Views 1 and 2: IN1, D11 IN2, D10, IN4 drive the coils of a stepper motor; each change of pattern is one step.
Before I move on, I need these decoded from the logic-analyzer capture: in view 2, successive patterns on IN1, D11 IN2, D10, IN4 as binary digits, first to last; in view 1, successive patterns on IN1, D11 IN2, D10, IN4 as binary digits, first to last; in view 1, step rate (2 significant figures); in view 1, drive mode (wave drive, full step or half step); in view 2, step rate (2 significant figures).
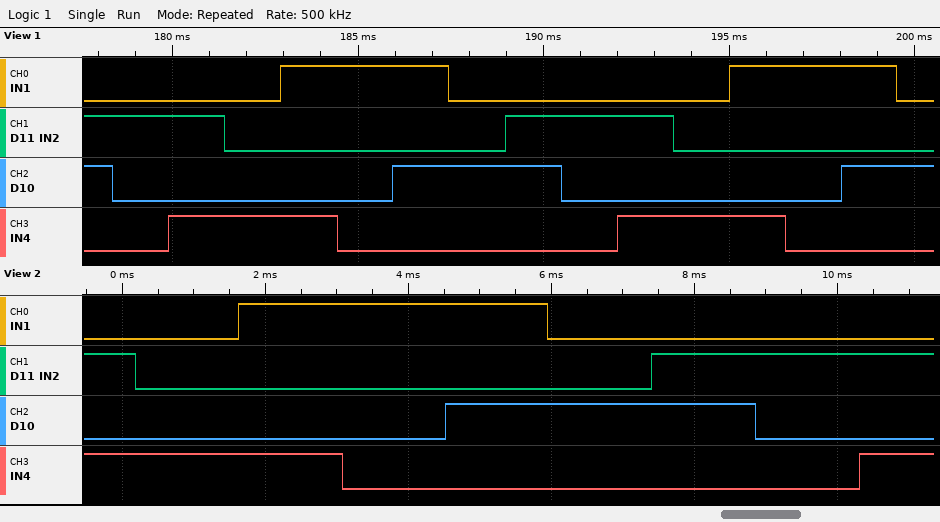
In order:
0101 0001 1001 1000 1010 0010 0110 0100 0101
0110 0100 0101 0001 1001 1000 1010 0010 0110 0100 0101 0001 1001 1000 1010 0010
660 steps/s
half step
690 steps/s
